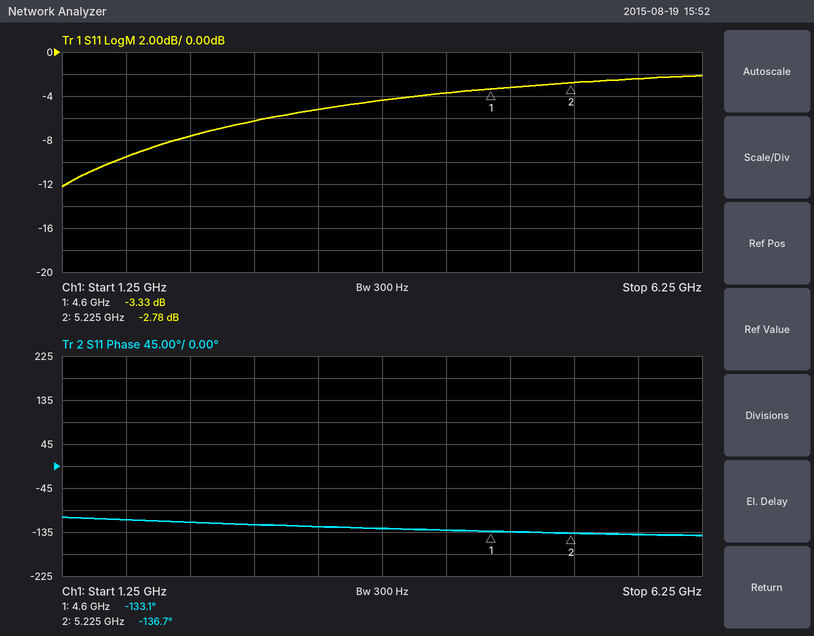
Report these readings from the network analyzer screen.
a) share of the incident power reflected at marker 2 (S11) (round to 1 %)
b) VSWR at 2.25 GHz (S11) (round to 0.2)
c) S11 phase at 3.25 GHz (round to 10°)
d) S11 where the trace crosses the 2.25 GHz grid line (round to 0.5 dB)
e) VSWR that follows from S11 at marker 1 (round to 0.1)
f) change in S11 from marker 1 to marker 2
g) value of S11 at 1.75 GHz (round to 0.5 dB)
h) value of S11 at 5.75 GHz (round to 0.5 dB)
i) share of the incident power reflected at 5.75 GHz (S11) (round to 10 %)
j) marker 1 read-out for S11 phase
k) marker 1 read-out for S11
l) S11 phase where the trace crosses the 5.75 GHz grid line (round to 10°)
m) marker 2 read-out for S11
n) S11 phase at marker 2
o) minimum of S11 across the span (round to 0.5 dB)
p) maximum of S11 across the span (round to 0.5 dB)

53 %
2.4
-120°
-7.5 dB
5.3
0.55 dB
-9.5 dB
-2.5 dB
60 %
-133.1°
-3.33 dB
-140°
-2.78 dB
-136.7°
-12.0 dB
-2.0 dB
